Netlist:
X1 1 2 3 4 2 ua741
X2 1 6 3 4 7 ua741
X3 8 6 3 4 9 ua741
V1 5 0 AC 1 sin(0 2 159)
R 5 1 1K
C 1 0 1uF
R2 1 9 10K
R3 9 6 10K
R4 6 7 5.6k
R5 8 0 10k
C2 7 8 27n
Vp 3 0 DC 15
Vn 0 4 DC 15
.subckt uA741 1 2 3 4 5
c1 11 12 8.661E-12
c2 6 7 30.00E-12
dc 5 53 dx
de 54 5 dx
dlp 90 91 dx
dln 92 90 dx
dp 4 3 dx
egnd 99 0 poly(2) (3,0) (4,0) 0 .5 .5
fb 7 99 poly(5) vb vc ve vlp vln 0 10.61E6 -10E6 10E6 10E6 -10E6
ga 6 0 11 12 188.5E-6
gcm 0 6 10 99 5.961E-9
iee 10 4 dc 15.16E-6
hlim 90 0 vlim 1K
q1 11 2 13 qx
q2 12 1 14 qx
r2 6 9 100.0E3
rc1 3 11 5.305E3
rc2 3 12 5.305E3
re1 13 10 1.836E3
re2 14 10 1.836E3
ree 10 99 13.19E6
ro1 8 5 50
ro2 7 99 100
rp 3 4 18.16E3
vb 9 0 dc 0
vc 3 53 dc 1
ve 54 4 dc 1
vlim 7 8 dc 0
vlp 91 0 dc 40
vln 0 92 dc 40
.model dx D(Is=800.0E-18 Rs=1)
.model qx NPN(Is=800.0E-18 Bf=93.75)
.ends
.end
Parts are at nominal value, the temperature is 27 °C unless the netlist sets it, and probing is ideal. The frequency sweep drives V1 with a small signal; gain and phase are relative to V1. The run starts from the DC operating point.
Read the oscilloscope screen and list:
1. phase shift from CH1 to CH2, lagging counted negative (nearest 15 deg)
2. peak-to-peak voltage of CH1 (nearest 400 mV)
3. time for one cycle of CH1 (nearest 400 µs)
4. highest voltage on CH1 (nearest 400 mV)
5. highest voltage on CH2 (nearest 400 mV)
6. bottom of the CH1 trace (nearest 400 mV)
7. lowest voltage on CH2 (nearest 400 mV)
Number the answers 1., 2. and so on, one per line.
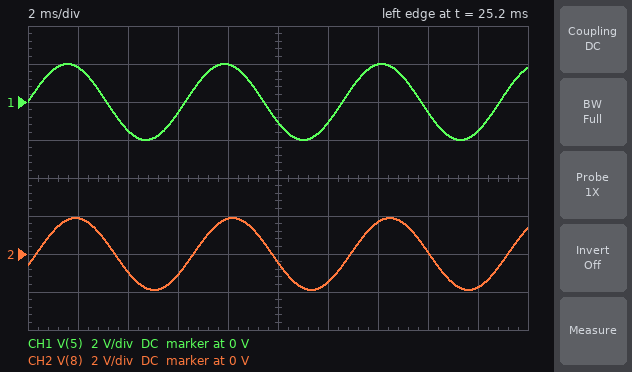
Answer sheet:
1. -15 deg
2. 4.0 V
3. 6.4 ms
4. 2.0 V
5. 2.0 V
6. -2.0 V
7. -2.0 V
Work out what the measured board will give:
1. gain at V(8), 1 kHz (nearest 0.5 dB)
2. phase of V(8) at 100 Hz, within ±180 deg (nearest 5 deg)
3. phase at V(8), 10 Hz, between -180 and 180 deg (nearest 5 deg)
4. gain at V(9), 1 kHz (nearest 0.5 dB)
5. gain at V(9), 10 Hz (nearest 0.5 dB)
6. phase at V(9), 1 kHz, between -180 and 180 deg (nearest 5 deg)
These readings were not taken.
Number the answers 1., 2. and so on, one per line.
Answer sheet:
1. -16.0 dB
2. 25 deg
3. 85 deg
4. -12.5 dB
5. 20.0 dB
6. -35 deg
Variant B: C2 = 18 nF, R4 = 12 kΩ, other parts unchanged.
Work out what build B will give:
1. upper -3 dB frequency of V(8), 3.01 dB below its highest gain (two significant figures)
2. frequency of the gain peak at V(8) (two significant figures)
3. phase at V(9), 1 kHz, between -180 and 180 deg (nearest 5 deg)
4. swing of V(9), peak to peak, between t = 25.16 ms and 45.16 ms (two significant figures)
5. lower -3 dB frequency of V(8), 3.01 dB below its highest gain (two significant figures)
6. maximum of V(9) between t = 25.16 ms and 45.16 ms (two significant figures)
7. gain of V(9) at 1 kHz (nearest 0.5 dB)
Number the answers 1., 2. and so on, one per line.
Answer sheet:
1. 210 Hz
2. 110 Hz
3. -45 deg
4. 17 V
5. 55 Hz
6. 8.3 V
7. -14.0 dB
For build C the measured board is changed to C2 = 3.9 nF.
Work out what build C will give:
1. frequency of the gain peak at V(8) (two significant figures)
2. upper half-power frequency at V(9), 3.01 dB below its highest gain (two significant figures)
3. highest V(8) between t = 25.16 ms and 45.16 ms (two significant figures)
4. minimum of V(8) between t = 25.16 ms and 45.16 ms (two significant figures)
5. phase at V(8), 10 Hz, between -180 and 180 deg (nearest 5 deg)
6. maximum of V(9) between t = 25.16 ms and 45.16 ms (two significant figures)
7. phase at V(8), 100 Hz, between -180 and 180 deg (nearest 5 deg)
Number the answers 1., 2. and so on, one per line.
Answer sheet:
1. 340 Hz
2. 390 Hz
3. 730 mV
4. -730 mV
5. 90 deg
6. 15 V
7. 80 deg
